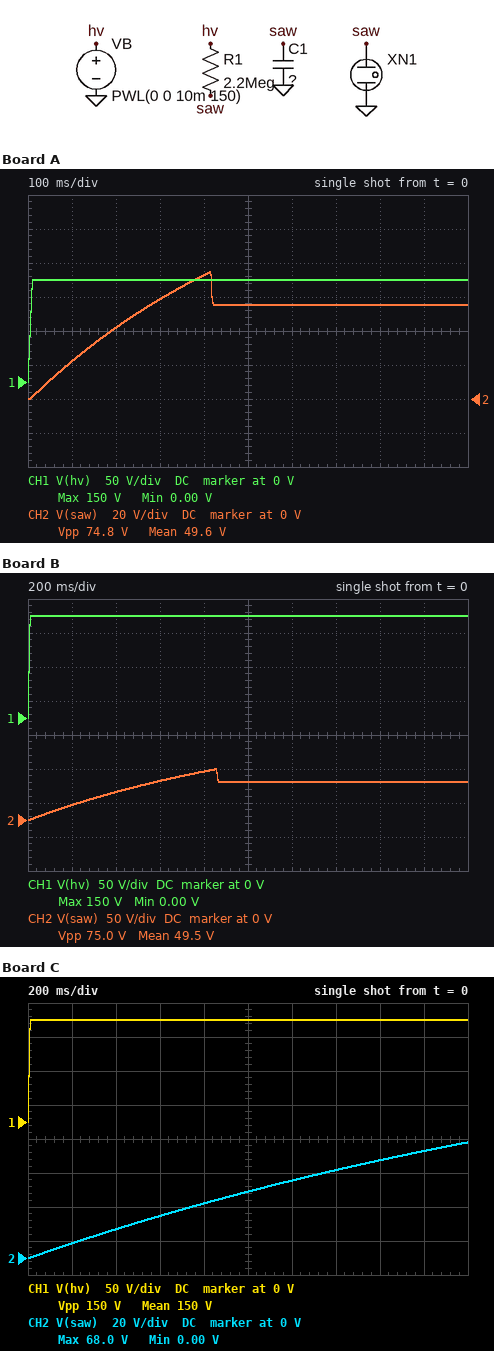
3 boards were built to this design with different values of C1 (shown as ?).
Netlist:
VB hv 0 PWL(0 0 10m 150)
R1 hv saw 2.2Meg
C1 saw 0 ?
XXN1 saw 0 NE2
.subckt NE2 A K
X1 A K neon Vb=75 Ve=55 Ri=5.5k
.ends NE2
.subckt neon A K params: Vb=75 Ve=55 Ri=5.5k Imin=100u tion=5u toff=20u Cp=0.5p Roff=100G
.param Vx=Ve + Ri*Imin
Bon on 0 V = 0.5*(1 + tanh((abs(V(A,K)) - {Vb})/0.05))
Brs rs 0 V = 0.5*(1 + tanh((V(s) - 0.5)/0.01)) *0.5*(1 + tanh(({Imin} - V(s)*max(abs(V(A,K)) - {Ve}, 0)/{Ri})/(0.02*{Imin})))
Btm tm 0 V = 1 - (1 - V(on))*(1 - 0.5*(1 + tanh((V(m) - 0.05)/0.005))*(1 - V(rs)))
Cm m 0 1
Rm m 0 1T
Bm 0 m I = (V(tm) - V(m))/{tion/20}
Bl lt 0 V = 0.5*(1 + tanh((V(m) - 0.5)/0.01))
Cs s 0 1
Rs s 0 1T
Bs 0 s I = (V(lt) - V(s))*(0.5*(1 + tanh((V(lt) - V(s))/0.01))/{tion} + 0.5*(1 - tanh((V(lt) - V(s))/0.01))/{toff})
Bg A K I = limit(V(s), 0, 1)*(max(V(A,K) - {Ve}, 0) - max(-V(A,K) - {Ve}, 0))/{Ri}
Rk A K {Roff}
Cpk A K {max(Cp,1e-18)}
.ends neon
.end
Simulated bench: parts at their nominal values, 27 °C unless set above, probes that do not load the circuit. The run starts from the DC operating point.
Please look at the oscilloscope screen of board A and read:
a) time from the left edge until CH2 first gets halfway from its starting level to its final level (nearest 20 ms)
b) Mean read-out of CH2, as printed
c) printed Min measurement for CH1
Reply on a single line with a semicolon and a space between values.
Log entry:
120 ms; 49.6 V; 0.00 V
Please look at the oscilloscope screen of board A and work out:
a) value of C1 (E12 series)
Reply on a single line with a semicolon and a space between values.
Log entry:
270 nF
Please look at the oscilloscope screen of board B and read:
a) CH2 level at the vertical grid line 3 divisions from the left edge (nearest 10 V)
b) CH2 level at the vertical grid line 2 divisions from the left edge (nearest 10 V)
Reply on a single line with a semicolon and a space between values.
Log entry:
60 V; 40 V
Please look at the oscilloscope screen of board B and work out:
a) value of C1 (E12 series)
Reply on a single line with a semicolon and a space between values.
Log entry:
560 nF
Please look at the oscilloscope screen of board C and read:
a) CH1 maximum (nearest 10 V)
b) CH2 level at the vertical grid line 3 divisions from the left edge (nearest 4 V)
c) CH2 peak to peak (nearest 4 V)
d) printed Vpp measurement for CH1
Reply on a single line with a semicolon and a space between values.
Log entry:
150 V; 24 V; 68 V; 150 V
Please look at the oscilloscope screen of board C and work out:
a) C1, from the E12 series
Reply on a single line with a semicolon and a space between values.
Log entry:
1.5 µF
